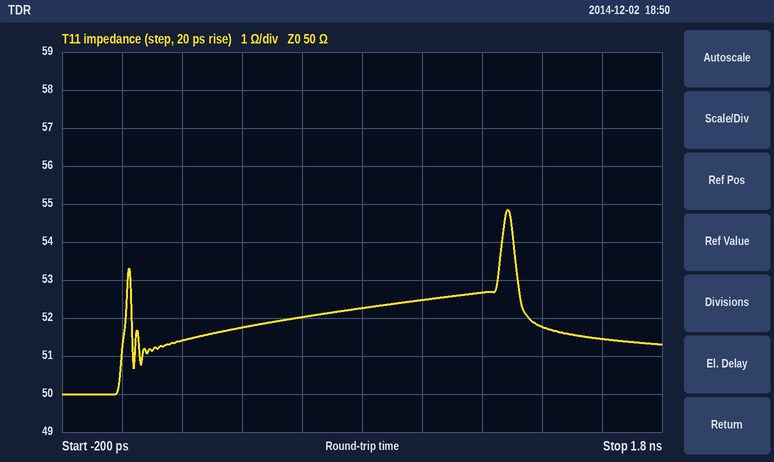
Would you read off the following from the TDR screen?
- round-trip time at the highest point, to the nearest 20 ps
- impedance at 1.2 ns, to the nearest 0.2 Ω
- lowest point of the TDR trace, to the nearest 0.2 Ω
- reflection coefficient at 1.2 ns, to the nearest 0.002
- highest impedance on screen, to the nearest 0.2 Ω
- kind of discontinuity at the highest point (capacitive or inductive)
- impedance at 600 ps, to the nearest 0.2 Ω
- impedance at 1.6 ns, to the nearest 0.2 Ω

1.28 ns
52.6 Ω
50.0 Ω
+0.026
54.8 Ω
inductive
52.0 Ω
51.4 Ω
